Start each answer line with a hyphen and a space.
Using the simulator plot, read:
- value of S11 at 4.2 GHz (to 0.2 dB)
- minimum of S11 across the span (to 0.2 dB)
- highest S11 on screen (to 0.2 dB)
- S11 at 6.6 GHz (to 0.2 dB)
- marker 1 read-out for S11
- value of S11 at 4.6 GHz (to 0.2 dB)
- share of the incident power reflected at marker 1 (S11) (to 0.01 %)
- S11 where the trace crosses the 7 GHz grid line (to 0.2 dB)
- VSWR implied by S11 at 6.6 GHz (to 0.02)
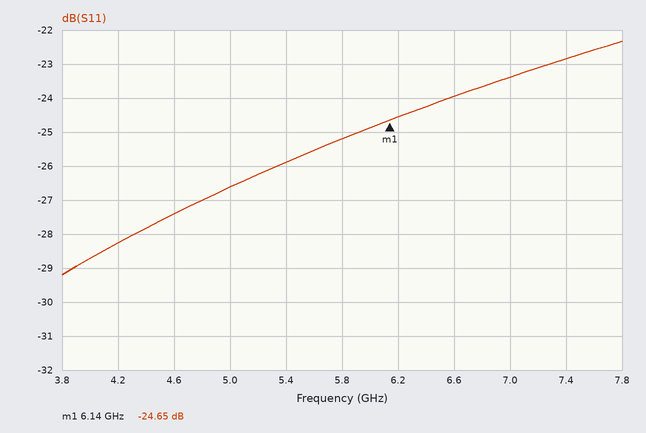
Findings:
- -28.2 dB
- -29.2 dB
- -22.4 dB
- -24.0 dB
- -24.65 dB
- -27.4 dB
- 0.34 %
- -23.4 dB
- 1.14
